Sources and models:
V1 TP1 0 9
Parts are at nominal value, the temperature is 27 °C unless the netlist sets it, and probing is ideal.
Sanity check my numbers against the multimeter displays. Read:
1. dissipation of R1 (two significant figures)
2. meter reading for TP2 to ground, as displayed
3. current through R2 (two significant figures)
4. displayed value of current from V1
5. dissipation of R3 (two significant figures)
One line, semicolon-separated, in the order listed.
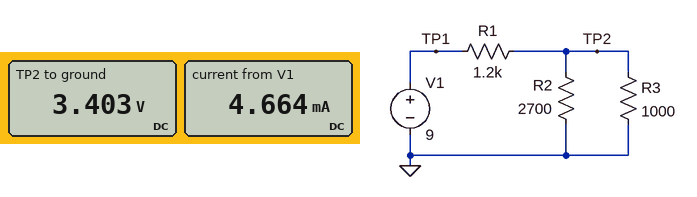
26 mW; 3.403 V; 1.3 mA; 4.664 mA; 12 mW
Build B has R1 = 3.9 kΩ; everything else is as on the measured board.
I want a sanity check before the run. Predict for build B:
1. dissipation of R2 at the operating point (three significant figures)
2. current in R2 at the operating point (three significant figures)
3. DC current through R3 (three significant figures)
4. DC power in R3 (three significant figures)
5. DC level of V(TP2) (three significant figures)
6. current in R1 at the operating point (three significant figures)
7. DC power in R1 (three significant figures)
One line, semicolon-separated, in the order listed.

745 µW; 525 µA; 1.42 mA; 2.01 mW; 1.42 V; 1.94 mA; 14.7 mW
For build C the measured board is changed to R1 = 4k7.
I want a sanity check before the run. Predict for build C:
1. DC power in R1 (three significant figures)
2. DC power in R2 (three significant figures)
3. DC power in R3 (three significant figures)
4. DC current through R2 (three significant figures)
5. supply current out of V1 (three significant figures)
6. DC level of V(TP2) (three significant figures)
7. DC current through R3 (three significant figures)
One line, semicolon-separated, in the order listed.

12.9 mW; 542 µW; 1.46 mW; 448 µA; 1.66 mA; 1.21 V; 1.21 mA
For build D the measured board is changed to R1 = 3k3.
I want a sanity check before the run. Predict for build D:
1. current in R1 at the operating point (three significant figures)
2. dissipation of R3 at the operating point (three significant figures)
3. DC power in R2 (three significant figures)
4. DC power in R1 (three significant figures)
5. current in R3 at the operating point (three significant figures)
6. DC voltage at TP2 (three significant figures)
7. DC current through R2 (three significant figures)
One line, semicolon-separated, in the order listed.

2.23 mA; 2.66 mW; 984 µW; 16.5 mW; 1.63 mA; 1.63 V; 604 µA
